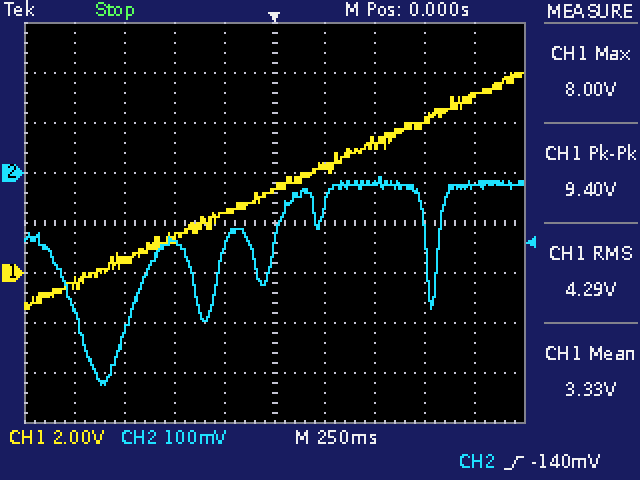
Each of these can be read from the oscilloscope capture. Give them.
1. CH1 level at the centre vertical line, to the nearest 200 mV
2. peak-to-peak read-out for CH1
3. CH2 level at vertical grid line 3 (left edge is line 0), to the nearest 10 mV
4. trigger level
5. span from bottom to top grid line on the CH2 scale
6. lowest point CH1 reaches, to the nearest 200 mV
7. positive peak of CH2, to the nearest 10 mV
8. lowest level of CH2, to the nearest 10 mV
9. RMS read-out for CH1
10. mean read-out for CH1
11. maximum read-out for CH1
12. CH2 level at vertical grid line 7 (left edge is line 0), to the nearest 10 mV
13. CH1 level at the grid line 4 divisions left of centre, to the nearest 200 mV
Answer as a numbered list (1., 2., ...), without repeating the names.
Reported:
1. 3.4 V
2. 9.40 V
3. -140 mV
4. -140 mV
5. 800 mV
6. -1.4 V
7. -10 mV
8. -420 mV
9. 4.29 V
10. 3.33 V
11. 8.00 V
12. -20 mV
13. -400 mV
